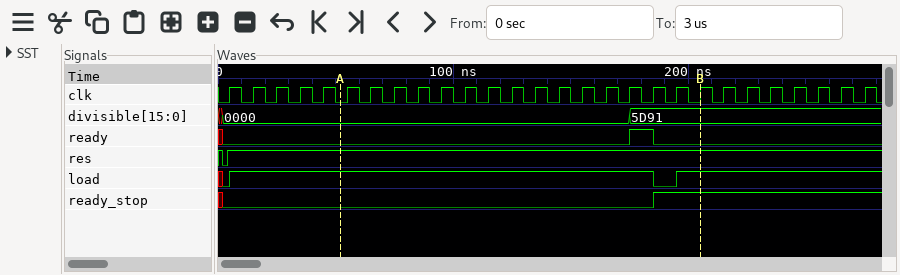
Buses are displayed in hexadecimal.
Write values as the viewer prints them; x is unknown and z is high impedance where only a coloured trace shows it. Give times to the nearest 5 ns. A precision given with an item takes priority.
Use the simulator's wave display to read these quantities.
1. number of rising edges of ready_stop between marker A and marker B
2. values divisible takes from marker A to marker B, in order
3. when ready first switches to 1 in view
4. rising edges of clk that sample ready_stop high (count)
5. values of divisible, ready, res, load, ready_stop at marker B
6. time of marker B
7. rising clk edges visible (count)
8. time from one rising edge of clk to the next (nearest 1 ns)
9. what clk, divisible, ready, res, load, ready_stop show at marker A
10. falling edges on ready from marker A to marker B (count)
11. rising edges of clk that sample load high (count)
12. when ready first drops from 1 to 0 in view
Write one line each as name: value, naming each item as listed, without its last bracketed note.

number of rising edges of ready_stop between marker A and marker B: 1
values divisible takes from marker A to marker B, in order: 0000, 5D91
when ready first switches to 1 in view: 175 ns
rising edges of clk that sample ready_stop high: 9
values of divisible, ready, res, load, ready_stop at marker B: divisible=5D91, ready=0, res=1, load=1, ready_stop=1
time of marker B: 205 ns
rising clk edges visible: 28
time from one rising edge of clk to the next: 10 ns
what clk, divisible, ready, res, load, ready_stop show at marker A: clk=0, divisible=0000, ready=0, res=1, load=1, ready_stop=0
falling edges on ready from marker A to marker B: 1
rising edges of clk that sample load high: 26
when ready first drops from 1 to 0 in view: 185 ns
